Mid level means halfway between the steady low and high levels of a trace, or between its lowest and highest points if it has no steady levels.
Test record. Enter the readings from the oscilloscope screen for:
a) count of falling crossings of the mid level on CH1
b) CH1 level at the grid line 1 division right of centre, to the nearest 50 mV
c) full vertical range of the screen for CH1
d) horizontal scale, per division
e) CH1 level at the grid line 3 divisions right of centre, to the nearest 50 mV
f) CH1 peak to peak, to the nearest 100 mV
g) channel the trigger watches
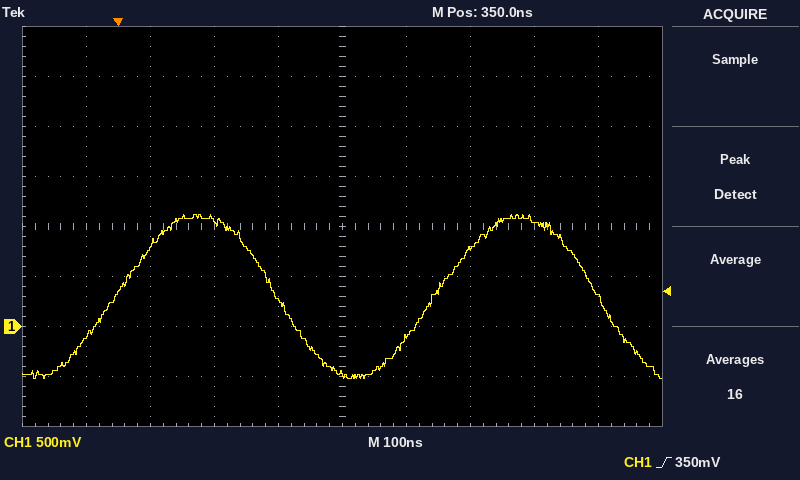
2
-100 mV
4 V
100 ns
1.05 V
1.60 V
CH1
